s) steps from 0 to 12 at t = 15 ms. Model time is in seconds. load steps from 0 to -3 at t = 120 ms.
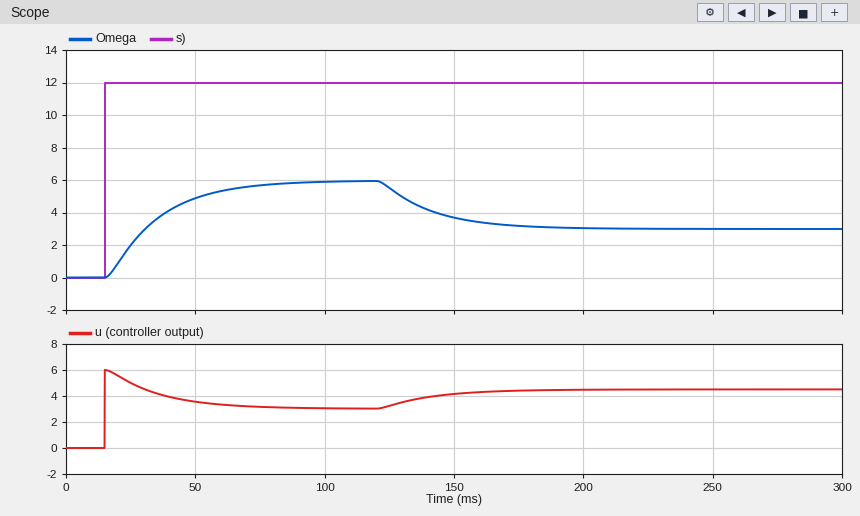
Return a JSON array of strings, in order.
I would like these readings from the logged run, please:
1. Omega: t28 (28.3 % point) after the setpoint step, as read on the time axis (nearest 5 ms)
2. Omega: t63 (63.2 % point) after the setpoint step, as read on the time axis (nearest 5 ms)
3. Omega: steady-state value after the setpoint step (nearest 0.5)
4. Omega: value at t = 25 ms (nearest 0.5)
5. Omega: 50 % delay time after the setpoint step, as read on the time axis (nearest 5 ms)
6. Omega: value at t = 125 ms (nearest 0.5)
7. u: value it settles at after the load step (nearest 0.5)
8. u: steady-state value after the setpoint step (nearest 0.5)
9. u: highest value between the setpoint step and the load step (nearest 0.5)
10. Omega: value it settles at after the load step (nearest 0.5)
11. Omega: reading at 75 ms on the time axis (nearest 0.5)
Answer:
["25 ms", "35 ms", "6.0", "2.0", "30 ms", "5.5", "4.5", "3.0", "6.0", "3.0", "5.5"]
